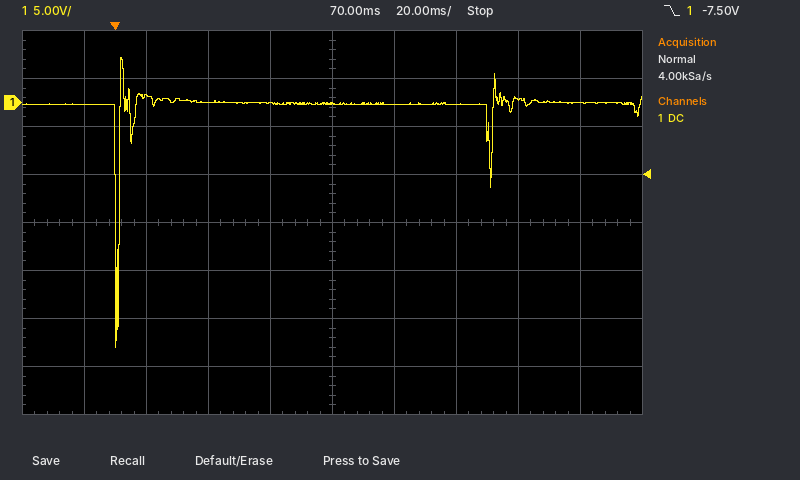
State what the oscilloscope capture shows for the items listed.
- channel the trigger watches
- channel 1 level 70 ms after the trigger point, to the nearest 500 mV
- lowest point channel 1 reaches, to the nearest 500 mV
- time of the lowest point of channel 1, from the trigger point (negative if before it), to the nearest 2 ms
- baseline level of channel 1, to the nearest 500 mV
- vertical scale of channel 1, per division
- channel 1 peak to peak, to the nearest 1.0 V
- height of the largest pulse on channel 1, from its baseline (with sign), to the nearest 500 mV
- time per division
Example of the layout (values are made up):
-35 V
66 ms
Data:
channel 1
0.0 V
-25.5 V
0 ms
0.0 V
5 V
30.0 V
-25.5 V
20 ms
